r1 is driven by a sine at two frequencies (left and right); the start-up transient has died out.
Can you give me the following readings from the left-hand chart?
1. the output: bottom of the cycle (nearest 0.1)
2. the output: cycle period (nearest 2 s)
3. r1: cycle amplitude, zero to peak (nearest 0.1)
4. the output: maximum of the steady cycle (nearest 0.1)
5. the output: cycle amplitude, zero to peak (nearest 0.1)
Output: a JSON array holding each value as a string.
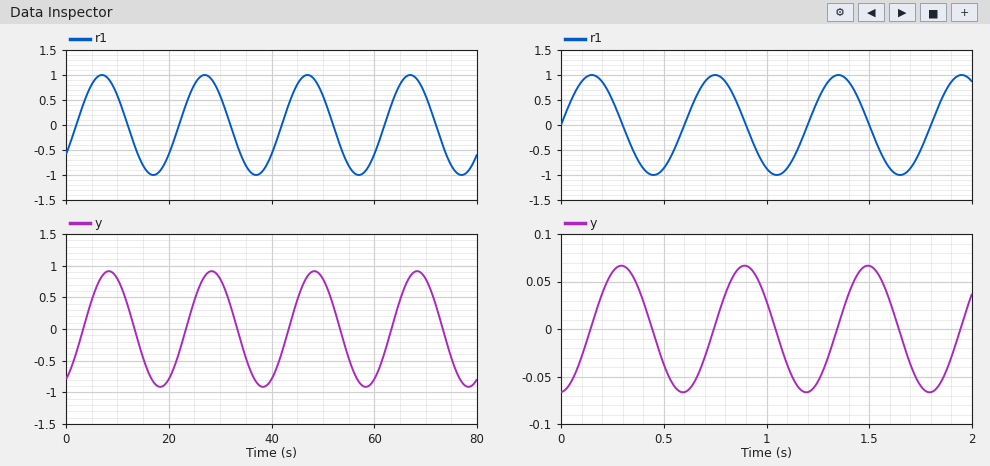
["-0.9", "20 s", "1.0", "0.9", "0.9"]
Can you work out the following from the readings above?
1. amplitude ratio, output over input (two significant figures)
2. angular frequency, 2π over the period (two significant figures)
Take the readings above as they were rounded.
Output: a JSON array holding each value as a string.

["0.90", "0.31 rad/s"]
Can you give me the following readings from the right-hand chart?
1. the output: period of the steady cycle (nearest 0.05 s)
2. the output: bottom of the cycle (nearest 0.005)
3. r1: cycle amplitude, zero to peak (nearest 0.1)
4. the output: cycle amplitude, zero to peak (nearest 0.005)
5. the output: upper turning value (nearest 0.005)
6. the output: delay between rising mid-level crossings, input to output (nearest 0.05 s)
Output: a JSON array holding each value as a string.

["0.60 s", "-0.065", "1.0", "0.065", "0.065", "0.15 s"]
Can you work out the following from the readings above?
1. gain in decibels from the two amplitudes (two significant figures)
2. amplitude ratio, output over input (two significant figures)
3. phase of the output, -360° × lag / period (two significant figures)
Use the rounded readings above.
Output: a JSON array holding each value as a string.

["-24 dB", "0.065", "-90°"]
